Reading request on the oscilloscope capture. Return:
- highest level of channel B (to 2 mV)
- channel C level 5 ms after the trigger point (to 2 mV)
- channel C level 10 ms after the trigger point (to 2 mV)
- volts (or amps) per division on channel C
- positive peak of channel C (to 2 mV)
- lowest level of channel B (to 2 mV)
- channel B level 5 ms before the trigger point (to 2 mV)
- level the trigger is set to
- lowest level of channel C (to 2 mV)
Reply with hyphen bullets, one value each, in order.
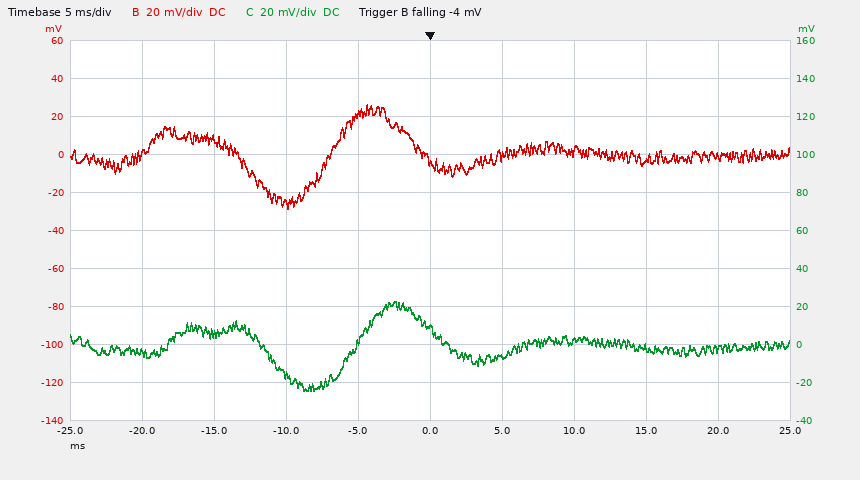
- 26 mV
- -6 mV
- 2 mV
- 20 mV
- 22 mV
- -28 mV
- 22 mV
- -4 mV
- -24 mV
